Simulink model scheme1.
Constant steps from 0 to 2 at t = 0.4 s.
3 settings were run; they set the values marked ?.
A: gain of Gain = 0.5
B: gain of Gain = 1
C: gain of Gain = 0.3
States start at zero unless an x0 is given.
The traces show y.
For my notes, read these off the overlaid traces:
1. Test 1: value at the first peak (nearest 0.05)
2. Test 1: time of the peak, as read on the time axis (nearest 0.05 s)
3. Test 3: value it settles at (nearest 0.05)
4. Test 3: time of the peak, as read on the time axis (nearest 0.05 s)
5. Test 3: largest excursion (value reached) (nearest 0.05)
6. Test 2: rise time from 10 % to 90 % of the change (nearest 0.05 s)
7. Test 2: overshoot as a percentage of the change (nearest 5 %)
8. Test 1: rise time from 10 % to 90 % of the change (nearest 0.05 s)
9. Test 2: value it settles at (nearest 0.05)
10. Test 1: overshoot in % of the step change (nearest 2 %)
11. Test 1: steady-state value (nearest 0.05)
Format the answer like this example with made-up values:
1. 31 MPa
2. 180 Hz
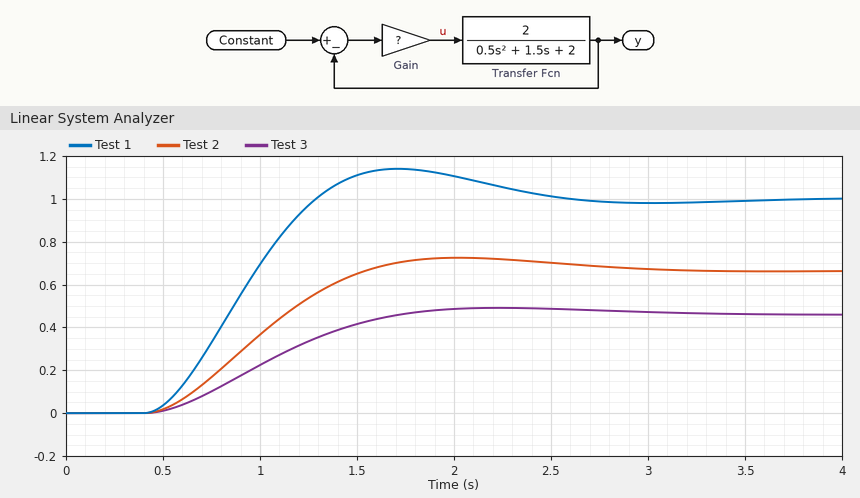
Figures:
1. 1.15
2. 1.70 s
3. 0.45
4. 2.25 s
5. 0.50
6. 0.75 s
7. 10 %
8. 0.60 s
9. 0.65
10. 14 %
11. 1.00
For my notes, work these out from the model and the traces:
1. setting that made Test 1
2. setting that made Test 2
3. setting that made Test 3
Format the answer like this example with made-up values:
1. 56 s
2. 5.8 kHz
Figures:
1. B
2. A
3. C
